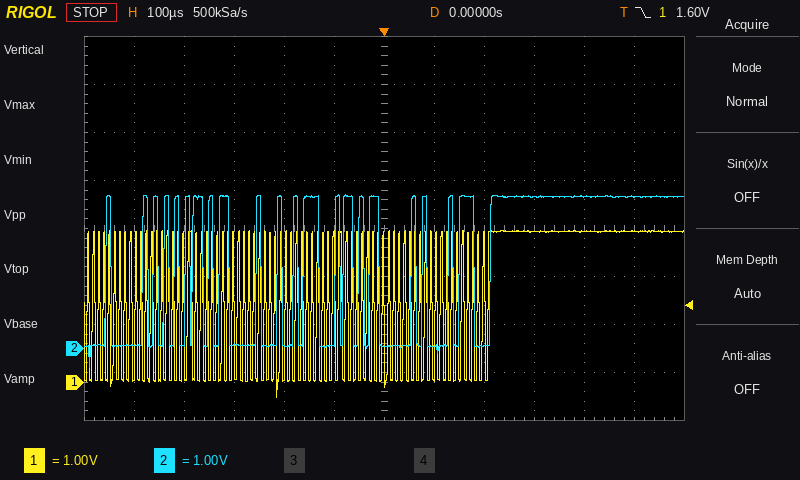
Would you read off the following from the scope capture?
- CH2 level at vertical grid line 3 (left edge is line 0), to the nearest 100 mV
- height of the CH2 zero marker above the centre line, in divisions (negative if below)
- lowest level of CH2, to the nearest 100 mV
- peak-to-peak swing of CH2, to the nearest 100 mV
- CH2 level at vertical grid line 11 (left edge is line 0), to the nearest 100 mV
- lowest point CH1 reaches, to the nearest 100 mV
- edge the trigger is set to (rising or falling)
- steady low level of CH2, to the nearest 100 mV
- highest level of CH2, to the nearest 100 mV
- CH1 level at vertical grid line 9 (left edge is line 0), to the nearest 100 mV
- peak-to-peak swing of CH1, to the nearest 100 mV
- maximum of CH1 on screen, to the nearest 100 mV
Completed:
100 mV
-2.5 div
-400 mV
3.6 V
3.2 V
-300 mV
falling
100 mV
3.2 V
3.1 V
3.5 V
3.2 V
